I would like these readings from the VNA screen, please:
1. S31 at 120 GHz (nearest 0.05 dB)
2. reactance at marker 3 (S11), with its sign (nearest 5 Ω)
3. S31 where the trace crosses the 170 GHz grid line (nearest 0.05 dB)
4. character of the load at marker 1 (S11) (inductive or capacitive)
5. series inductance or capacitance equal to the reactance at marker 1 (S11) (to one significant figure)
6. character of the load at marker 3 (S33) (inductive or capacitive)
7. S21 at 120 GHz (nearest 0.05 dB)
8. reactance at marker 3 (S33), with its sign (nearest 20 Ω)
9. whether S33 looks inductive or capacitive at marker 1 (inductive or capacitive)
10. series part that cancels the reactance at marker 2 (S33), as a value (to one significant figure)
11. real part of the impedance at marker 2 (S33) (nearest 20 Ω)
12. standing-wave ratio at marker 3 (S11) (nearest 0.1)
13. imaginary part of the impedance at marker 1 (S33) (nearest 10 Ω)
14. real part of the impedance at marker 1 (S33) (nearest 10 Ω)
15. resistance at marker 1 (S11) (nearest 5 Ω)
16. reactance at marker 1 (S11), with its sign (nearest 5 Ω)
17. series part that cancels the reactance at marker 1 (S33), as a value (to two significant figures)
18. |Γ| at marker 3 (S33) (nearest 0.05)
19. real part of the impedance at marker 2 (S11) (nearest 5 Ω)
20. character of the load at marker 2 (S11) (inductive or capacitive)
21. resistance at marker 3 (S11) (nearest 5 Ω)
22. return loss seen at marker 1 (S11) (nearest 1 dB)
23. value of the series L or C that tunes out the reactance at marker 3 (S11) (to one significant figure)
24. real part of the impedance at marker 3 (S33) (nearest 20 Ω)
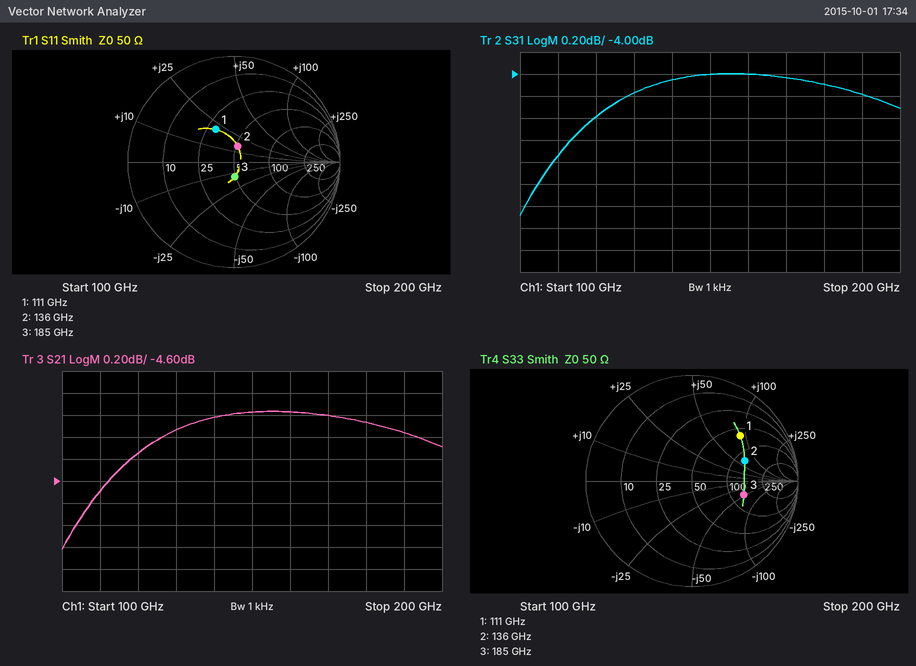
-4.40 dB
-15 Ω
-4.05 dB
inductive
30 pH
capacitive
-4.35 dB
-40 Ω
inductive
20 fF
120 Ω
1.3
+90 Ω
60 Ω
30 Ω
+20 Ω
16 fF
0.50
50 Ω
inductive
50 Ω
9 dB
10 pH
140 Ω
